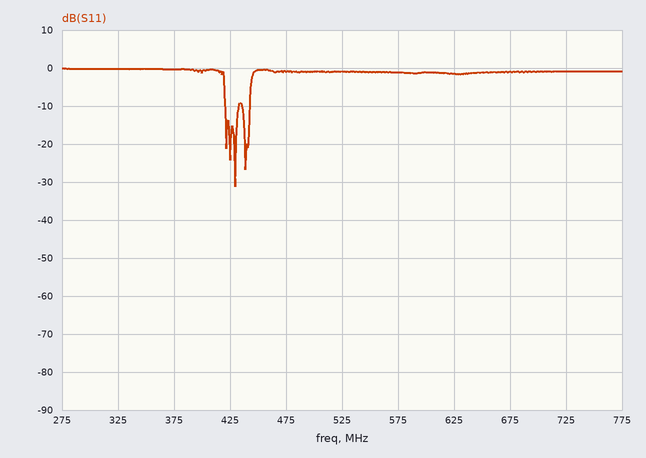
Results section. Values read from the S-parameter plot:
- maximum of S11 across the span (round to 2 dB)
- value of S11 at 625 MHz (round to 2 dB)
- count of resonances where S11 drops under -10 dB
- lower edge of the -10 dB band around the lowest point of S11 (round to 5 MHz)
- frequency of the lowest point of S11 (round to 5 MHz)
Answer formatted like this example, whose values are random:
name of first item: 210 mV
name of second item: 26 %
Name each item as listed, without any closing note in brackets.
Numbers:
maximum of S11 across the span: 0 dB
value of S11 at 625 MHz: -2 dB
count of resonances where S11 drops under -10 dB: 4
lower edge of the -10 dB band around the lowest point of S11: 420 MHz
frequency of the lowest point of S11: 430 MHz
